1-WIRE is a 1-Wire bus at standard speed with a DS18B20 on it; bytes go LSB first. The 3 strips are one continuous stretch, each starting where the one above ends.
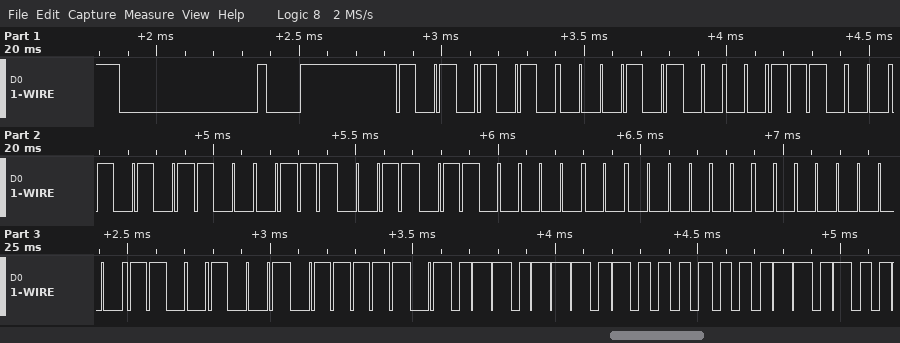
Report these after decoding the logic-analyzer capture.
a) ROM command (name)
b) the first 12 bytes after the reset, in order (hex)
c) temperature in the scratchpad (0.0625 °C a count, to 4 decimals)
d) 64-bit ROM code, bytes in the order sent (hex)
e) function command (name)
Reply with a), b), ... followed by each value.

a) Match ROM
b) 55 28 1C 35 CE 06 00 00 93 BE 76 01
c) 23.3750 °C
d) 28 1C 35 CE 06 00 00 93
e) Read Scratchpad
